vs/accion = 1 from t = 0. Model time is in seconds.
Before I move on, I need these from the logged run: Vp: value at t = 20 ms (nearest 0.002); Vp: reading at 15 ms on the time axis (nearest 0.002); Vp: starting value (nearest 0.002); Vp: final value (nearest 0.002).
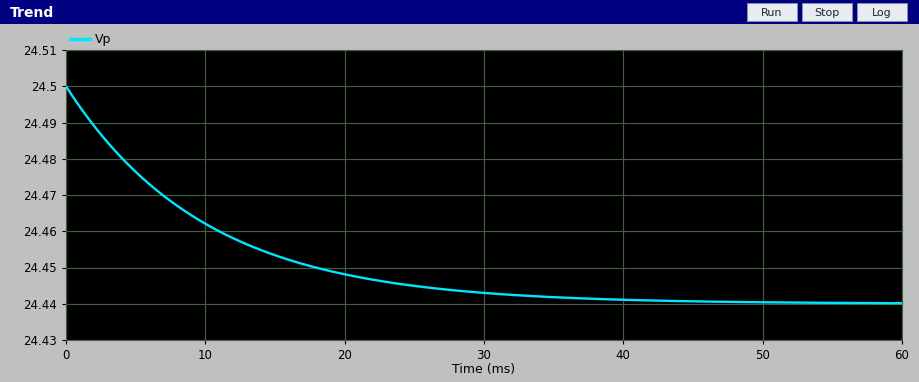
24.448
24.454
24.500
24.440
